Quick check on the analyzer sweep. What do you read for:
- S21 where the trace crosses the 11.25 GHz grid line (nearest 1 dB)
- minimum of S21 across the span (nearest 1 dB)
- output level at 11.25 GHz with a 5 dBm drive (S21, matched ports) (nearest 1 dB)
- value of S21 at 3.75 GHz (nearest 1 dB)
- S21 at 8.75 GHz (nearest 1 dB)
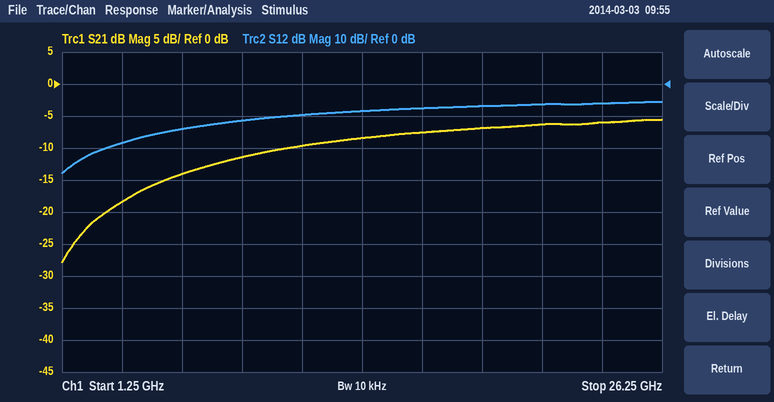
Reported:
-10 dB
-28 dB
-5 dBm
-18 dB
-11 dB
